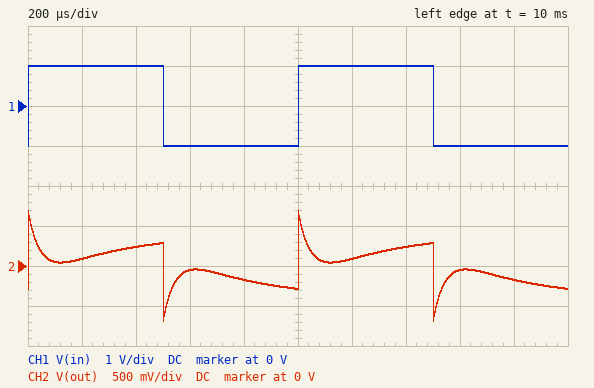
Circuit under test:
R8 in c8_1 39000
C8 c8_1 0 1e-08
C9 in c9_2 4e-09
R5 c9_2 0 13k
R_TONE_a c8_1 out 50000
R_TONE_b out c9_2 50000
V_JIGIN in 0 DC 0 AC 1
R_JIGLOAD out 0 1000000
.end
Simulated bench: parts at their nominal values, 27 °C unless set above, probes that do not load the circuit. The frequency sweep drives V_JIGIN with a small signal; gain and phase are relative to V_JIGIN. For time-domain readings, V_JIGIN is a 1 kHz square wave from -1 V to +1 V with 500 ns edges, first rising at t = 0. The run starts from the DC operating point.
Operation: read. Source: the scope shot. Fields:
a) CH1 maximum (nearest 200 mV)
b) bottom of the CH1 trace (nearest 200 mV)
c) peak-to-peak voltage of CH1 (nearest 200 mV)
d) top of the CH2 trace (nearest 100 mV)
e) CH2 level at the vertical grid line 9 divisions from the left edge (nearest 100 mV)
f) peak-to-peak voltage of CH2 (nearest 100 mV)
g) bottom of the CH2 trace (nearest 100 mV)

1.0 V
-1.0 V
2.0 V
700 mV
-200 mV
1.4 V
-700 mV
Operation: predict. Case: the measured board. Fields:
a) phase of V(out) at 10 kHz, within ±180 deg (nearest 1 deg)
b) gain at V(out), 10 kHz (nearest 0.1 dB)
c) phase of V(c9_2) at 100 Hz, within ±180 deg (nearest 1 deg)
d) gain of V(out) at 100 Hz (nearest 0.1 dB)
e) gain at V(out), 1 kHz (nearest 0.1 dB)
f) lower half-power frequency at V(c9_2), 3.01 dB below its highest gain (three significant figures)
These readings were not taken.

16 deg
-6.8 dB
9 deg
-8.1 dB
-16.5 dB
3.57 kHz
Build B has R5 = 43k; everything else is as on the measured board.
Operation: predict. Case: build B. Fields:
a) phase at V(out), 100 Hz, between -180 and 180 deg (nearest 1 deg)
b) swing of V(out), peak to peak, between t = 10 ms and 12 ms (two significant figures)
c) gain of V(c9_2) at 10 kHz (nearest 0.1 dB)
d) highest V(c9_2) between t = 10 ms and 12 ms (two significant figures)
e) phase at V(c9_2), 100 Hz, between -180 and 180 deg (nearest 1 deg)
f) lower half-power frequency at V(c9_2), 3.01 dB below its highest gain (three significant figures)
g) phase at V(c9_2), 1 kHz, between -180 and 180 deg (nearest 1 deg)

-6 deg
1.2 V
-0.1 dB
1.8 V
6 deg
1.55 kHz
47 deg
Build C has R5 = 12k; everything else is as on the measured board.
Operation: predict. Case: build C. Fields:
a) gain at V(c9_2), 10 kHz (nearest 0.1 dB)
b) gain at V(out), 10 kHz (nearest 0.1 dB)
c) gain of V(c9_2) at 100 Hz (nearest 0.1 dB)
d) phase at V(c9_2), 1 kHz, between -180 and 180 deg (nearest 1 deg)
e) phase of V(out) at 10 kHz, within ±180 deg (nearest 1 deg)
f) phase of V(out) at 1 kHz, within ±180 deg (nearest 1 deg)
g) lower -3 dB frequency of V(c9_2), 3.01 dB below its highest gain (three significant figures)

-0.6 dB
-6.9 dB
-22.4 dB
70 deg
17 deg
-17 deg
3.82 kHz
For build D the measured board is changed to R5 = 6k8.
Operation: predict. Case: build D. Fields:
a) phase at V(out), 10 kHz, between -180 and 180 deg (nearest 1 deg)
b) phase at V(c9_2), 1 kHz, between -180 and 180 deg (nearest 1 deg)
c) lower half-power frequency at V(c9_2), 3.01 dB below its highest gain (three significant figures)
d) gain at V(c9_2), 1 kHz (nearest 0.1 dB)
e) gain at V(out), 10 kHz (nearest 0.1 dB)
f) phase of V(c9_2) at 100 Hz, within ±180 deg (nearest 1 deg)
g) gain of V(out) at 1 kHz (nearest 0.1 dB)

29 deg
76 deg
6.32 kHz
-17.1 dB
-7.9 dB
10 deg
-17.2 dB
